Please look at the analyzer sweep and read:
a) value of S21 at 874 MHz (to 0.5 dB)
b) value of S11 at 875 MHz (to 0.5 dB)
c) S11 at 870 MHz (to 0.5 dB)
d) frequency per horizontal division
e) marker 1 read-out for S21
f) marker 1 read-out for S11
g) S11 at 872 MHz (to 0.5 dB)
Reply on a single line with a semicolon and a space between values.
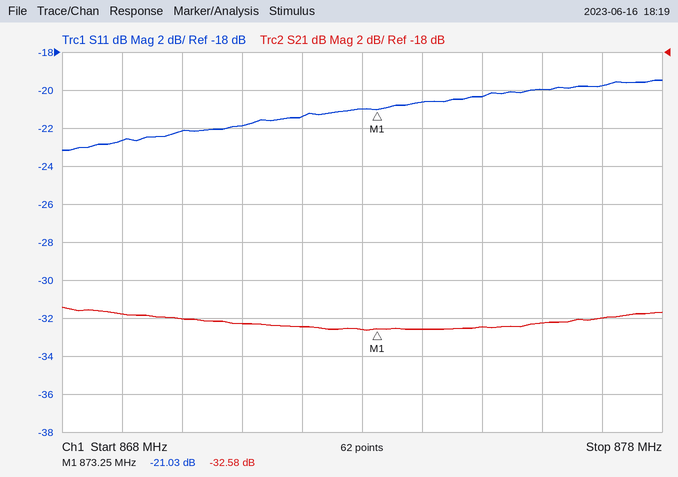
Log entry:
-32.5 dB; -20.5 dB; -22.0 dB; 1 MHz; -32.58 dB; -21.03 dB; -21.5 dB
